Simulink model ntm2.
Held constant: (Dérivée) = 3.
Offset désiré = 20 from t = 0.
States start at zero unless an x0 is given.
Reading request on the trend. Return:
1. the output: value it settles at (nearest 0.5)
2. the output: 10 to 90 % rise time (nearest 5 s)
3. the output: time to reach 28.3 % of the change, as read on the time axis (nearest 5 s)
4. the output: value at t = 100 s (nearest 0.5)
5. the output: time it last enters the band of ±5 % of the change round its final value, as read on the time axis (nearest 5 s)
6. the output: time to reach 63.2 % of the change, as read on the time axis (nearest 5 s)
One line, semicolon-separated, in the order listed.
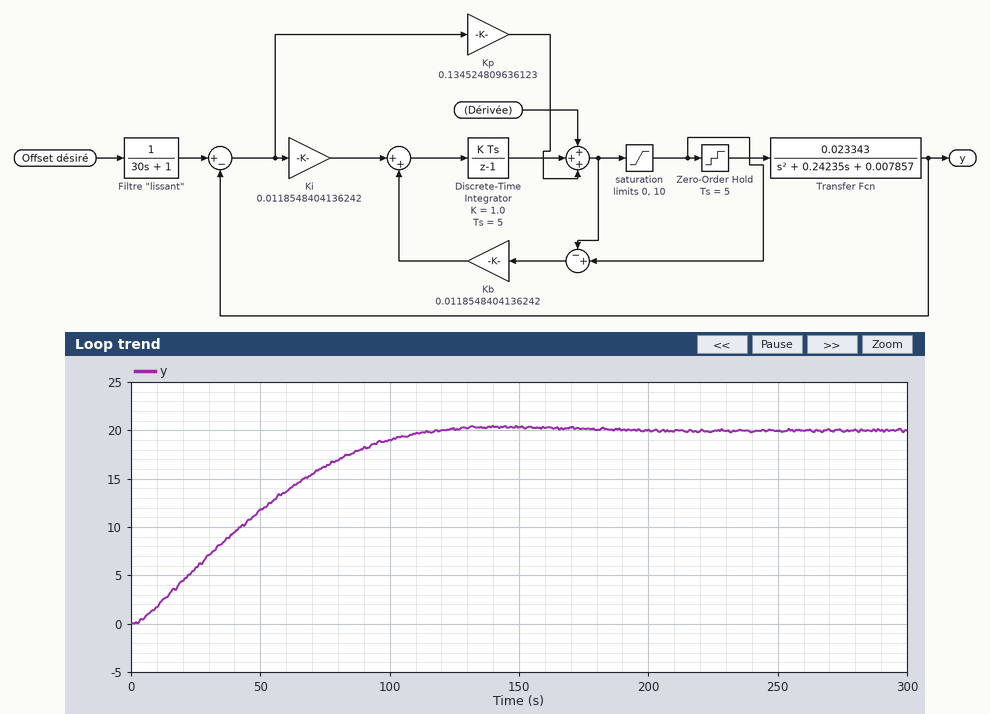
20.0; 80 s; 25 s; 19.0; 100 s; 55 s
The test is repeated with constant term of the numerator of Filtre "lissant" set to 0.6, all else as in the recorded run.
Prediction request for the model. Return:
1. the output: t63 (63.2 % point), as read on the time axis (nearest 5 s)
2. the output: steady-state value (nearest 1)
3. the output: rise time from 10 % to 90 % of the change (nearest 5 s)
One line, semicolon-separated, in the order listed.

40 s; 12; 70 s
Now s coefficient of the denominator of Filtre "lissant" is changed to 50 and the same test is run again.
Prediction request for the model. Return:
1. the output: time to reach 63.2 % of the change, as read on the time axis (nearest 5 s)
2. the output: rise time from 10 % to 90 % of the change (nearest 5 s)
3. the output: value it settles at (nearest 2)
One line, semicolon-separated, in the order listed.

75 s; 125 s; 20
